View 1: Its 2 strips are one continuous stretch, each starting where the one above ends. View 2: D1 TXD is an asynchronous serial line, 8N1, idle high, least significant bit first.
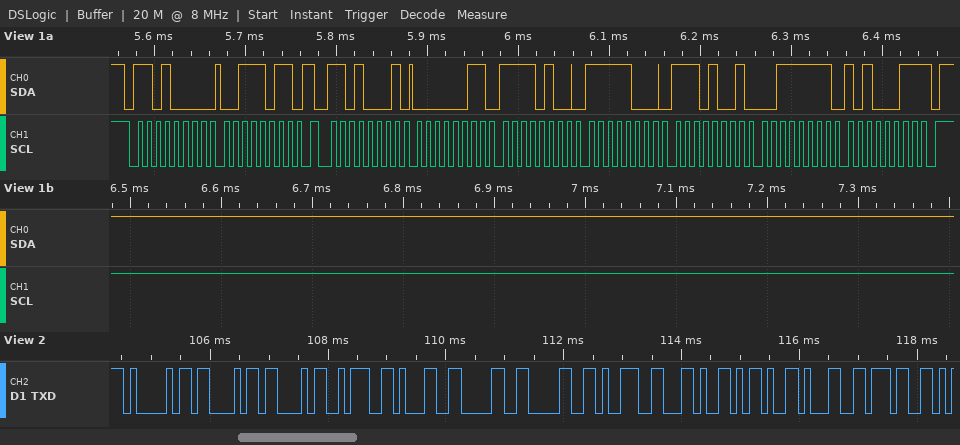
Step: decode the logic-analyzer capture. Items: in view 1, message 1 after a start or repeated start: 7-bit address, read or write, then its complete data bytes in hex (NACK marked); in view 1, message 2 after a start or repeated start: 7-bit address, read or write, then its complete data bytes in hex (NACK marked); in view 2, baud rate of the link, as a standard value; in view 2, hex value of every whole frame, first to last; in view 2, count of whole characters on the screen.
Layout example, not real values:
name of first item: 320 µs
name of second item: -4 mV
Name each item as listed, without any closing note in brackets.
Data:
in view 1, message 1 after a start or repeated start: 7-bit address, read or write, then its complete data bytes in hex: 0x68 write: 3B
in view 1, message 2 after a start or repeated start: 7-bit address, read or write, then its complete data bytes in hex: 0x68 read: 03 F4 F8 E9 3F A3 NACK
in view 2, baud rate of the link, as a standard value: 9600 baud
in view 2, hex value of every whole frame, first to last: 0x41 0x43 0x43 0x3A 0x31 0x30 0x30 0x39 0x2C 0x2D 0x31 0x37
in view 2, count of whole characters on the screen: 12
